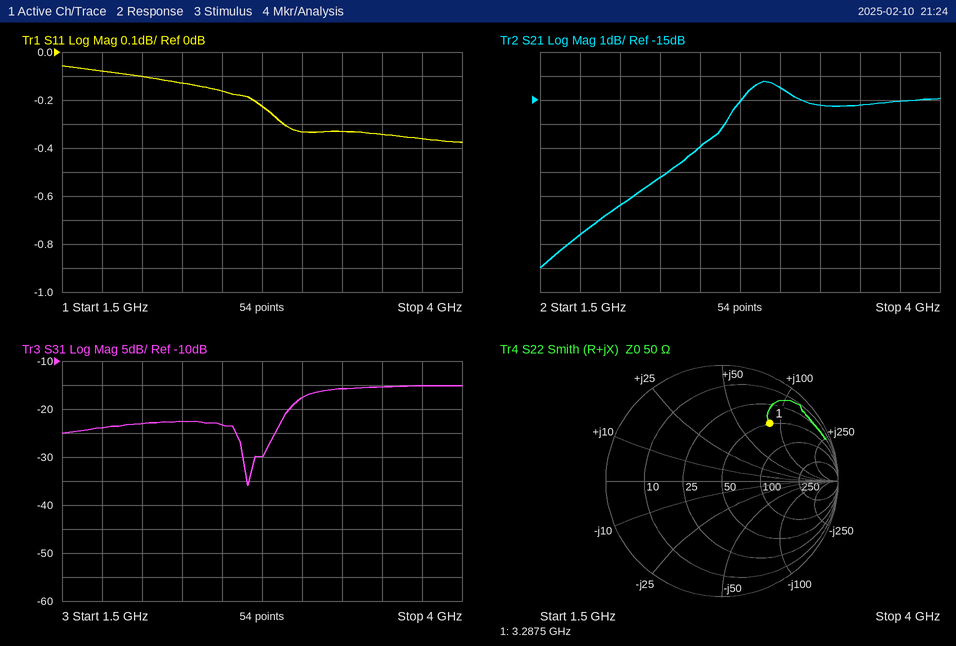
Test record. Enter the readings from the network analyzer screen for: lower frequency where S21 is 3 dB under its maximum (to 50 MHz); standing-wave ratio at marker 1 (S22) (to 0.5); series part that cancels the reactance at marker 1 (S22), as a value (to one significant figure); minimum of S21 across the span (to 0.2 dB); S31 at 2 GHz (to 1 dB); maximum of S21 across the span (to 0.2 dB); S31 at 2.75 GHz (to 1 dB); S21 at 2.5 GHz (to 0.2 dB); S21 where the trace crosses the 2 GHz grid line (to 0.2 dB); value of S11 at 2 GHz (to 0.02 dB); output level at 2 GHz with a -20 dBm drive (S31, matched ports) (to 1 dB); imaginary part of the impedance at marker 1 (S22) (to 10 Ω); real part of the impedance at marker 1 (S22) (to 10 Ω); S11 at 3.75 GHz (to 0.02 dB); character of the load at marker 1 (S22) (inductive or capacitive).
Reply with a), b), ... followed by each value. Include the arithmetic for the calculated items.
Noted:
a) 2.45 GHz
b) 4.5
c) C = 1/(2π × 3.2875 GHz × 80 Ω) ≈ 605 fF, so 600 fF to one significant figure
d) -22.0 dB
e) -23 dB
f) -14.2 dB
g) -30 dB
h) -17.0 dB
i) -19.4 dB
j) -0.10 dB
k) -20 dBm + (-23 dB) = -43 dBm
l) +80 Ω
m) 50 Ω
n) -0.36 dB
o) inductive
